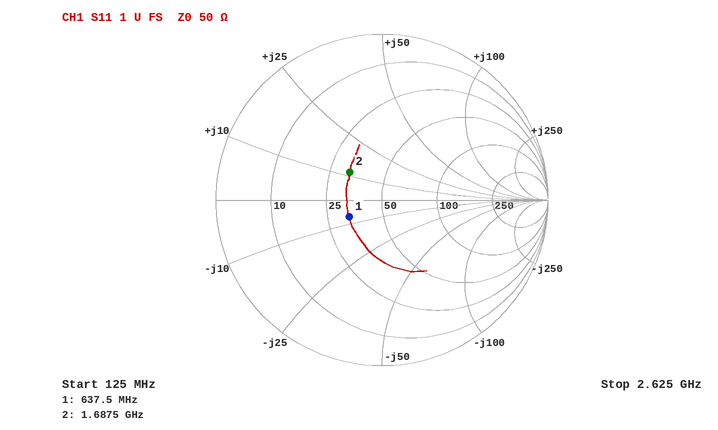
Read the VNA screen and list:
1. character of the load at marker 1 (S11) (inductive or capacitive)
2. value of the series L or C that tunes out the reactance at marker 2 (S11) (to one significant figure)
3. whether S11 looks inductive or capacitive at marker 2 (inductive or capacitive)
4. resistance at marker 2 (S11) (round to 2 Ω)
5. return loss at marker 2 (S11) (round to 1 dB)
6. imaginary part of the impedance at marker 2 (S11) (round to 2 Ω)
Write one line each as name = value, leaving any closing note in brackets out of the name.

character of the load at marker 1 (S11) = capacitive
value of the series L or C that tunes out the reactance at marker 2 (S11) = 8 pF
whether S11 looks inductive or capacitive at marker 2 = inductive
resistance at marker 2 (S11) = 32 Ω
return loss at marker 2 (S11) = 12 dB
imaginary part of the impedance at marker 2 (S11) = +12 Ω
